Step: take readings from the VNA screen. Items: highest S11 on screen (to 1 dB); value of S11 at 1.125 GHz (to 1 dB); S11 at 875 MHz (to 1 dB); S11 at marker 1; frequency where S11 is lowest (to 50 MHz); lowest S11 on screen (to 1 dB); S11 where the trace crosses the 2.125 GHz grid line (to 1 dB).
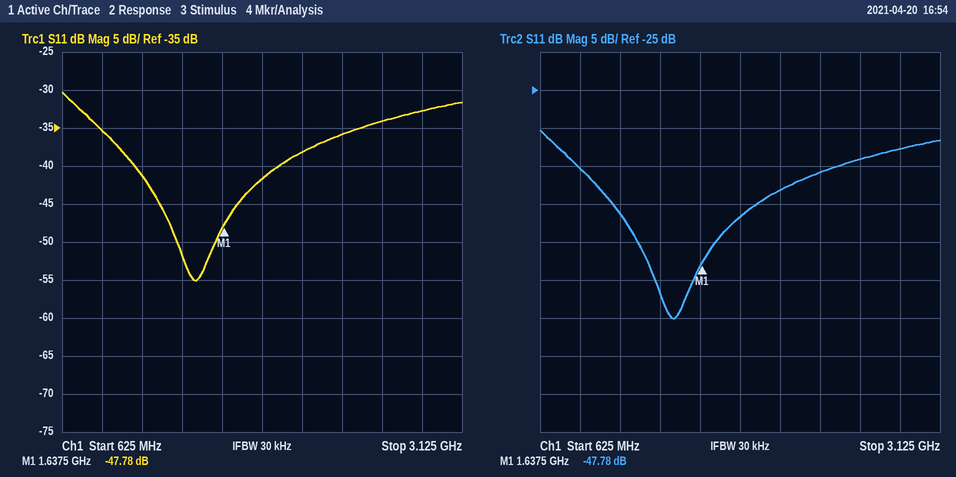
-30 dB
-41 dB
-35 dB
-47.78 dB
1.45 GHz
-55 dB
-38 dB
